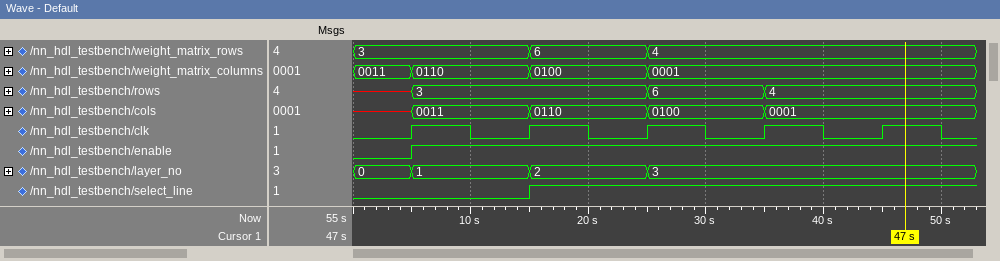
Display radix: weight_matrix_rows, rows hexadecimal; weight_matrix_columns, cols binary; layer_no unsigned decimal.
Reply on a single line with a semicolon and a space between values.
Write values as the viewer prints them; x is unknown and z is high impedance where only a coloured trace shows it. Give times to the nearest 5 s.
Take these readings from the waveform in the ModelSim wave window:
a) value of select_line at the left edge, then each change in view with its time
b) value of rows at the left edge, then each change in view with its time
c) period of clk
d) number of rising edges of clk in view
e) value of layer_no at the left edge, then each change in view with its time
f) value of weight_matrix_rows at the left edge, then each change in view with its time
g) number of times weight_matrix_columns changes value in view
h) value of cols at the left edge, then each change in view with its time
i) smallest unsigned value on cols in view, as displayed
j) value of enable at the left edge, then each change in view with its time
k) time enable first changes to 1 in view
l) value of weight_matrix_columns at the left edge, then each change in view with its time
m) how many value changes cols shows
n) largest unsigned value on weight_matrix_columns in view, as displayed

0, 1 at 15 s; x, 3 at 5 s, 6 at 25 s, 4 at 35 s; 10 s; 5; 0, 1 at 5 s, 2 at 15 s, 3 at 25 s; 3, 6 at 15 s, 4 at 25 s; 3; x, 0011 at 5 s, 0110 at 15 s, 0100 at 25 s, 0001 at 35 s; 0001; 0, 1 at 5 s; 5 s; 0011, 0110 at 5 s, 0100 at 15 s, 0001 at 25 s; 4; 0110
